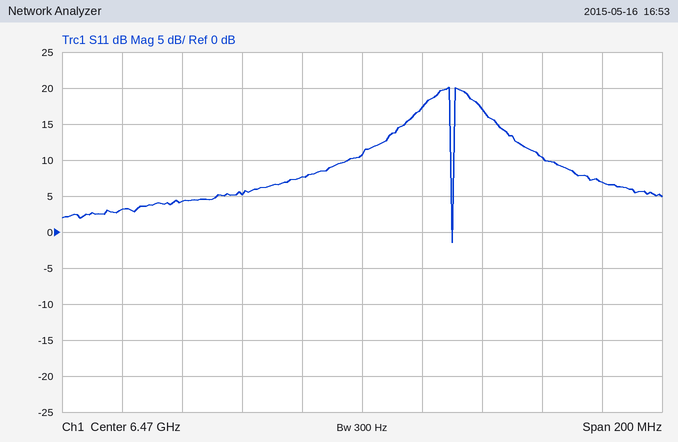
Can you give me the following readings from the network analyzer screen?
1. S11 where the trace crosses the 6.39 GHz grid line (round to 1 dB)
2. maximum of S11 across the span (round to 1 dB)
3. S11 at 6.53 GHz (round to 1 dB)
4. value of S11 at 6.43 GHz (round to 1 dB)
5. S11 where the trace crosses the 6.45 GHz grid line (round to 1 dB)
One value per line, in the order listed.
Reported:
3 dB
20 dB
10 dB
5 dB
8 dB
